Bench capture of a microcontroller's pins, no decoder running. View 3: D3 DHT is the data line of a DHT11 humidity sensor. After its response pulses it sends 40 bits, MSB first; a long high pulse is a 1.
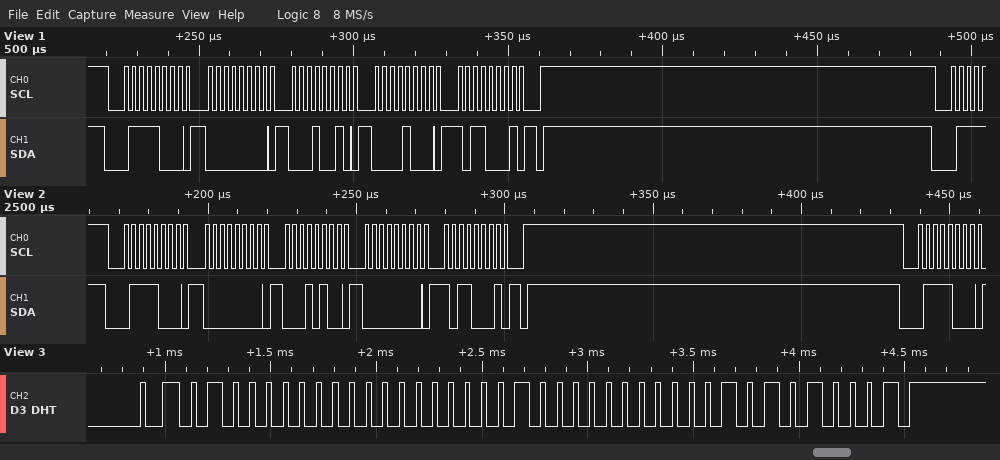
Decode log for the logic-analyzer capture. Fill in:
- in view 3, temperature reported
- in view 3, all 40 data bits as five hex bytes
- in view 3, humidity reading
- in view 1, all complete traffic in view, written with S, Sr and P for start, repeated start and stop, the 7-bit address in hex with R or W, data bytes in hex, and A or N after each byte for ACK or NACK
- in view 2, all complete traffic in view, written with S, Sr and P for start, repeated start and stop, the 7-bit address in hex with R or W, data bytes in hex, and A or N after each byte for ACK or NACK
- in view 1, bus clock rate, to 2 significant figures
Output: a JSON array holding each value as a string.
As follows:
["16.1 °C", "40 00 10 01 51", "64 %", "S 3CW A 00 A 12 A 08 A B1 A P", "S 3CW A 00 A 14 A 00 A B1 A P S 3CW A", "400 kHz"]
